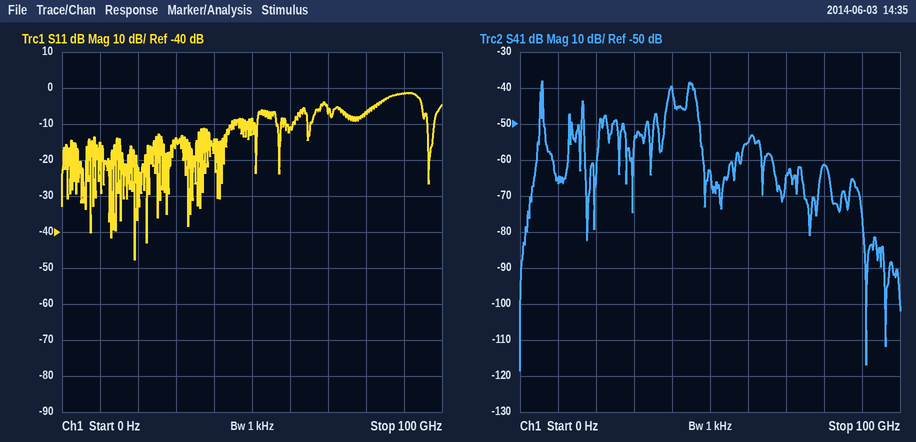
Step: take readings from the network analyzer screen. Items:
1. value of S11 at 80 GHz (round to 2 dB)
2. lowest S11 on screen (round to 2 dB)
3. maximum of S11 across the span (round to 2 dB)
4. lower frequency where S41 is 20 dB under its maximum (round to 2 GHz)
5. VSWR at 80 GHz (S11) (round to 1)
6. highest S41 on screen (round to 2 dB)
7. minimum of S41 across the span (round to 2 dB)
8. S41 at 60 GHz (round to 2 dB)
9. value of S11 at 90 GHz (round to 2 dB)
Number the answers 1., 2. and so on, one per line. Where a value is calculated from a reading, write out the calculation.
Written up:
1. -6 dB
2. -48 dB
3. -2 dB
4. 4 GHz
5. |Γ| = 10^(-6/20) = 0.5012; VSWR = (1 + 0.5012)/(1 − 0.5012) ≈ 3
6. -38 dB
7. -118 dB
8. -56 dB
9. -2 dB
